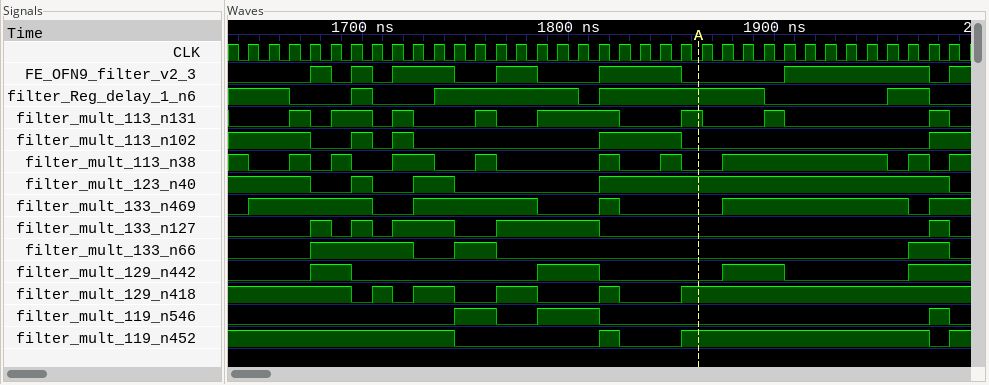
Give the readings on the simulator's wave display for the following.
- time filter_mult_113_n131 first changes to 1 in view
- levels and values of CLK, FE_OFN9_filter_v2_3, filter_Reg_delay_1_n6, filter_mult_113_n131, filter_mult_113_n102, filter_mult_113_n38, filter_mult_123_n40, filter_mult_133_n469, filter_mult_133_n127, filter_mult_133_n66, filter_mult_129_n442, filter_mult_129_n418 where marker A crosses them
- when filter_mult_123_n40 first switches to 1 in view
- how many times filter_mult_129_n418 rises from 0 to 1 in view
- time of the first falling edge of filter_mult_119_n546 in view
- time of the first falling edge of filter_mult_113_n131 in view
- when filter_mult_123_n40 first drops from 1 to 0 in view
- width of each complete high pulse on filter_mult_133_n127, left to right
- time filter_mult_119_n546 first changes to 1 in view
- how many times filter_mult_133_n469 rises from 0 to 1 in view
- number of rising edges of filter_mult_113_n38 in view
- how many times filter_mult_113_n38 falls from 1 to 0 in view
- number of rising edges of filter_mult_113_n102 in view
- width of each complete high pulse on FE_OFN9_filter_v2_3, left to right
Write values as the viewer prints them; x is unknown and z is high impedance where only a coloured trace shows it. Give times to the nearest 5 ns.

1665 ns
CLK=0, FE_OFN9_filter_v2_3=0, filter_Reg_delay_1_n6=1, filter_mult_113_n131=1, filter_mult_113_n102=0, filter_mult_113_n38=0, filter_mult_123_n40=1, filter_mult_133_n469=0, filter_mult_133_n127=0, filter_mult_133_n66=0, filter_mult_129_n442=0, filter_mult_129_n418=1
1695 ns
5
1765 ns
1675 ns
1675 ns
10 ns, 10 ns, 30 ns, 50 ns, 10 ns
1745 ns
5
9
9
4
10 ns, 10 ns, 30 ns, 20 ns, 40 ns, 70 ns
